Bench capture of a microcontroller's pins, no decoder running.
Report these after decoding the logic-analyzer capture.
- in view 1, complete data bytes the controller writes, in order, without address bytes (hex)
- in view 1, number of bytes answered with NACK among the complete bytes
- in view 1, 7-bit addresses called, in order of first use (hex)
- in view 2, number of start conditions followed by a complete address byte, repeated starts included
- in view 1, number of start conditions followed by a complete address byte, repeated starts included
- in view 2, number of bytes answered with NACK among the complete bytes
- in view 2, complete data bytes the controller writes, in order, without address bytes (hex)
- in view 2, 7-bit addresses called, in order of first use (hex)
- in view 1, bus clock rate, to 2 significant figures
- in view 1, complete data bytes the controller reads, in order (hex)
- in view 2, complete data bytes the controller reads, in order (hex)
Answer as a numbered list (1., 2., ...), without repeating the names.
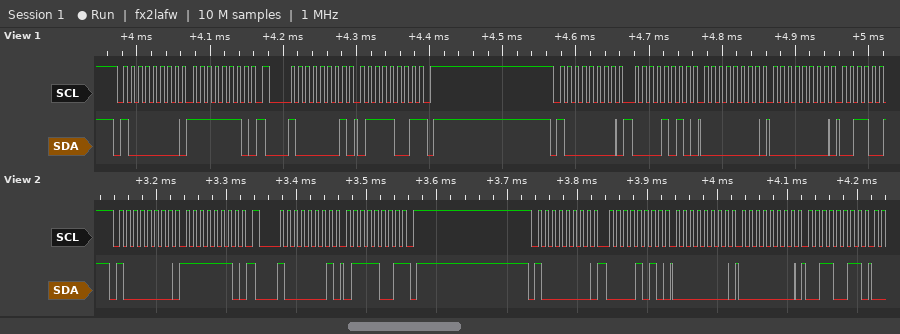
1. FE 0A 00 00
2. 1
3. 0x40
4. 3
5. 3
6. 1
7. FE 0A 00 00 33
8. 0x40
9. 100 kHz
10. 79
11. 79
